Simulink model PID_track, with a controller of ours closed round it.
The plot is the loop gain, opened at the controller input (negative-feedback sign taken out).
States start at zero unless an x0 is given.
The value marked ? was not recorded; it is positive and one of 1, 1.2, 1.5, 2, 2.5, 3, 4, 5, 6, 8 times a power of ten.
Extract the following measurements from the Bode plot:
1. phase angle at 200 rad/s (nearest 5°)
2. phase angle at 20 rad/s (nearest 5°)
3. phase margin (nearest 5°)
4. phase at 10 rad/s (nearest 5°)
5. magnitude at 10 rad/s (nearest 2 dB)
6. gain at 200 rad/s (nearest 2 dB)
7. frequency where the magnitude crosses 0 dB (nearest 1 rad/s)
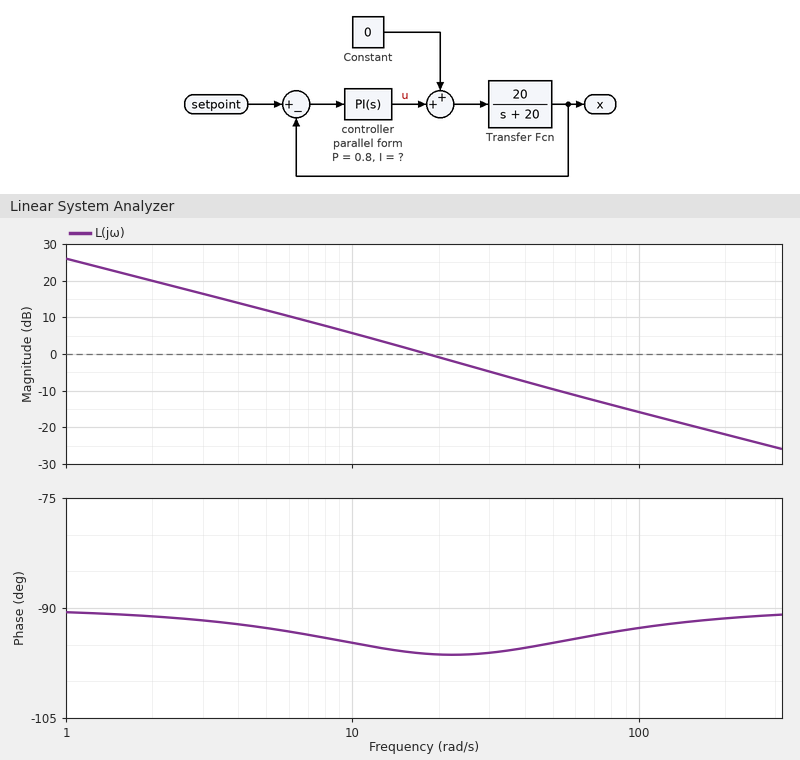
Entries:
-90°
-95°
85°
-95°
6 dB
-22 dB
18 rad/s
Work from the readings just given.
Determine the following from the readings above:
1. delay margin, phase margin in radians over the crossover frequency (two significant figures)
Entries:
0.082 s
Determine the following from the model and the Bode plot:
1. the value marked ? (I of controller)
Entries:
20
